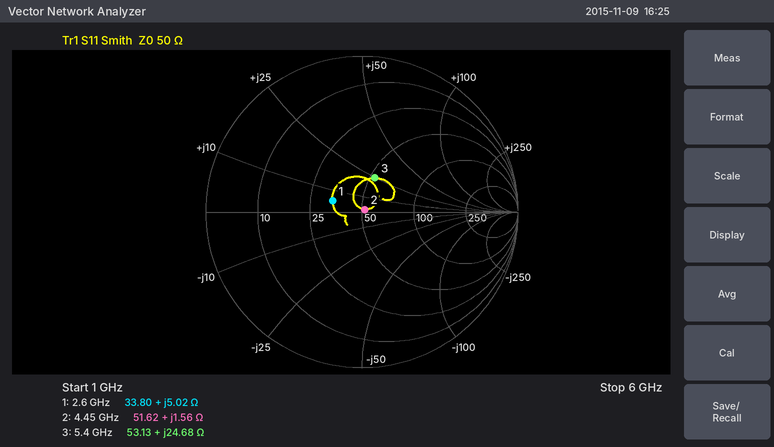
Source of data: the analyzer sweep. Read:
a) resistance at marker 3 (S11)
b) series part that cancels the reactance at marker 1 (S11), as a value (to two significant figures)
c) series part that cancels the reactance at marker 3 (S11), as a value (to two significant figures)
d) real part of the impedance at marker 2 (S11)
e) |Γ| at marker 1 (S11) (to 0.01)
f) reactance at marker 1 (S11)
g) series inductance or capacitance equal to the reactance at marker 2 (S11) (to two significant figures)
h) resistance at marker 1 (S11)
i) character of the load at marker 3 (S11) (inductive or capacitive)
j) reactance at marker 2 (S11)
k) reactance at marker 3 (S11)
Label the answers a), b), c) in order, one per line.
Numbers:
a) 53.13 Ω
b) 12 pF
c) 1.2 pF
d) 51.62 Ω
e) 0.20
f) +5.02 Ω
g) 56 pH
h) 33.80 Ω
i) inductive
j) +1.56 Ω
k) +24.68 Ω
